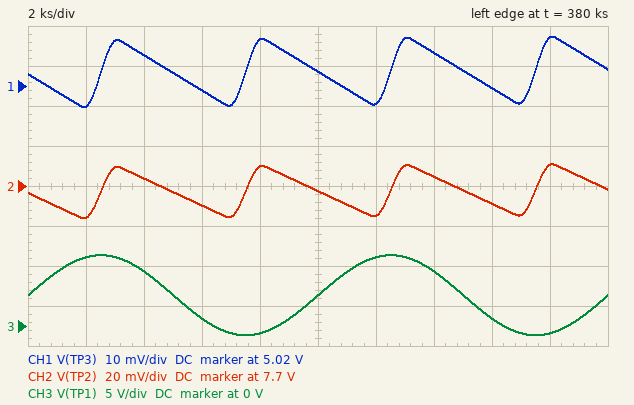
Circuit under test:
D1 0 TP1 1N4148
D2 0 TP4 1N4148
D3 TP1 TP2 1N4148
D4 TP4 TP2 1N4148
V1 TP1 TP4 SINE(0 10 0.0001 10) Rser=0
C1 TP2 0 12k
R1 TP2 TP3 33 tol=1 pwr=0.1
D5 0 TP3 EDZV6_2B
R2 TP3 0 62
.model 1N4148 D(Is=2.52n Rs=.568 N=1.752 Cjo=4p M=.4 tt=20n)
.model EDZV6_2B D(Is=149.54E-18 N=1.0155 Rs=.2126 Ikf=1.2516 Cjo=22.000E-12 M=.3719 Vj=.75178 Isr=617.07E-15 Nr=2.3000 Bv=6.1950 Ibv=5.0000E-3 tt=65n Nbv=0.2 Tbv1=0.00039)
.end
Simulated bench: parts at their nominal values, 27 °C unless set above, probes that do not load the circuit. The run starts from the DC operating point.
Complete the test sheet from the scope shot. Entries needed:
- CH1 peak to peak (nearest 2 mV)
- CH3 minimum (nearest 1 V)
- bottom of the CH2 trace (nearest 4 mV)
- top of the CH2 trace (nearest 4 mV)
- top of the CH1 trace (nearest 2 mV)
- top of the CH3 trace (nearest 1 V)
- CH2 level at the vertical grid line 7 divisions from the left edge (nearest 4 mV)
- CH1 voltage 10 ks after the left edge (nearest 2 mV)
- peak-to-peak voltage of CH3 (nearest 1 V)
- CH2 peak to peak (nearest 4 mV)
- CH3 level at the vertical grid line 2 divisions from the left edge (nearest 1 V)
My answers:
18 mV
-1 V
7.684 V
7.712 V
5.032 V
9 V
7.704 V
5.024 V
10 V
28 mV
7 V
